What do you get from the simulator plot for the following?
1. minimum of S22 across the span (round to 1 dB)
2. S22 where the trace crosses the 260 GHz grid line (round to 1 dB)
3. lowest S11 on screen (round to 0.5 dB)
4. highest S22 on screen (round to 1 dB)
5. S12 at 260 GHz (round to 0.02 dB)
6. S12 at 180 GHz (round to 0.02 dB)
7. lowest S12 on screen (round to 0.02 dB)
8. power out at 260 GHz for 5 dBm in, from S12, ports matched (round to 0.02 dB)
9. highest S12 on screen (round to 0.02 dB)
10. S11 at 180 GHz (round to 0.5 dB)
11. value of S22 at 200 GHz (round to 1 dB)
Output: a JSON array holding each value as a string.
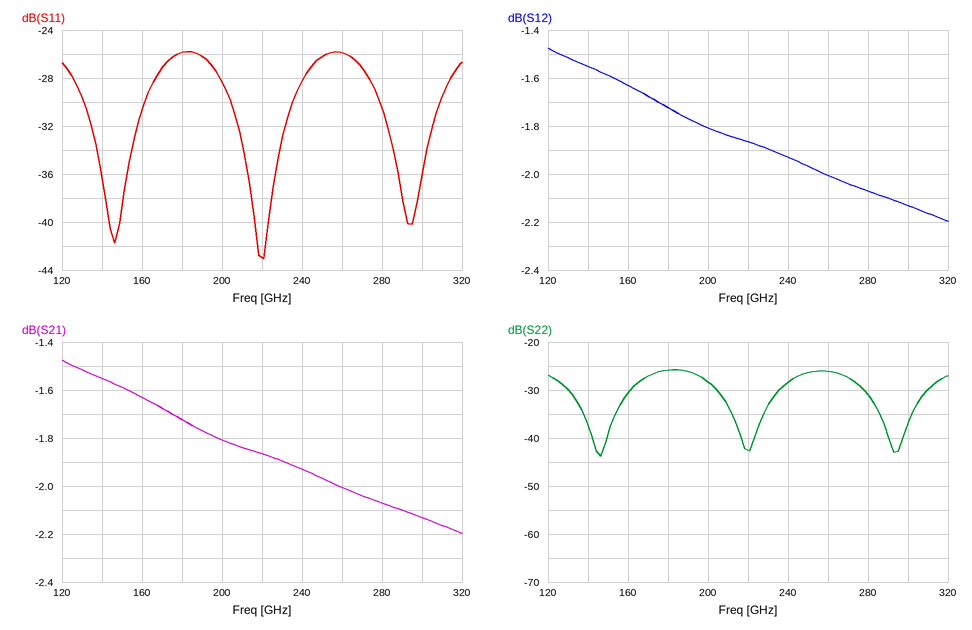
["-44 dB", "-26 dB", "-43.0 dB", "-26 dB", "-2.00 dB", "-1.72 dB", "-2.20 dB", "3.00 dBm", "-1.48 dB", "-26.0 dB", "-28 dB"]
